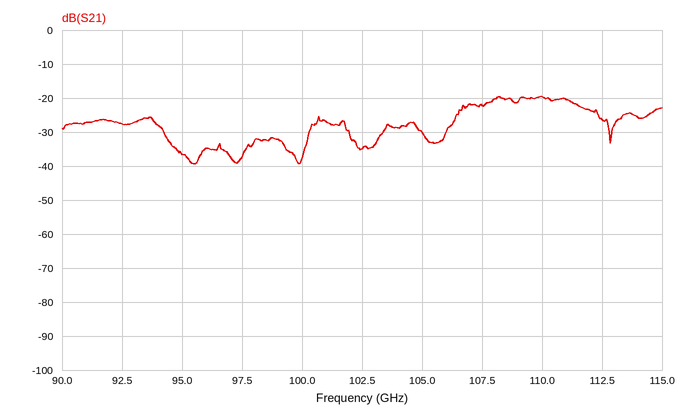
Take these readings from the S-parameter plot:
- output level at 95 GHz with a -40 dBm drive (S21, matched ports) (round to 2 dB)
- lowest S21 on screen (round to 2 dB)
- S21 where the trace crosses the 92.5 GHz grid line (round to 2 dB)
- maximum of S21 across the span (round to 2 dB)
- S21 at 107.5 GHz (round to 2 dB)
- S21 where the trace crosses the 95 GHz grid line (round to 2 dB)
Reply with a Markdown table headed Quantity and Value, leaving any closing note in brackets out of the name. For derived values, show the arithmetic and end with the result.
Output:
| Quantity | Value |
|---|---|
| output level at 95 GHz with a -40 dBm drive (S21, matched ports) | -40 dBm + (-36 dB) = -76 dBm |
| lowest S21 on screen | -40 dB |
| S21 where the trace crosses the 92.5 GHz grid line | -28 dB |
| maximum of S21 across the span | -20 dB |
| S21 at 107.5 GHz | -22 dB |
| S21 where the trace crosses the 95 GHz grid line | -36 dB |
